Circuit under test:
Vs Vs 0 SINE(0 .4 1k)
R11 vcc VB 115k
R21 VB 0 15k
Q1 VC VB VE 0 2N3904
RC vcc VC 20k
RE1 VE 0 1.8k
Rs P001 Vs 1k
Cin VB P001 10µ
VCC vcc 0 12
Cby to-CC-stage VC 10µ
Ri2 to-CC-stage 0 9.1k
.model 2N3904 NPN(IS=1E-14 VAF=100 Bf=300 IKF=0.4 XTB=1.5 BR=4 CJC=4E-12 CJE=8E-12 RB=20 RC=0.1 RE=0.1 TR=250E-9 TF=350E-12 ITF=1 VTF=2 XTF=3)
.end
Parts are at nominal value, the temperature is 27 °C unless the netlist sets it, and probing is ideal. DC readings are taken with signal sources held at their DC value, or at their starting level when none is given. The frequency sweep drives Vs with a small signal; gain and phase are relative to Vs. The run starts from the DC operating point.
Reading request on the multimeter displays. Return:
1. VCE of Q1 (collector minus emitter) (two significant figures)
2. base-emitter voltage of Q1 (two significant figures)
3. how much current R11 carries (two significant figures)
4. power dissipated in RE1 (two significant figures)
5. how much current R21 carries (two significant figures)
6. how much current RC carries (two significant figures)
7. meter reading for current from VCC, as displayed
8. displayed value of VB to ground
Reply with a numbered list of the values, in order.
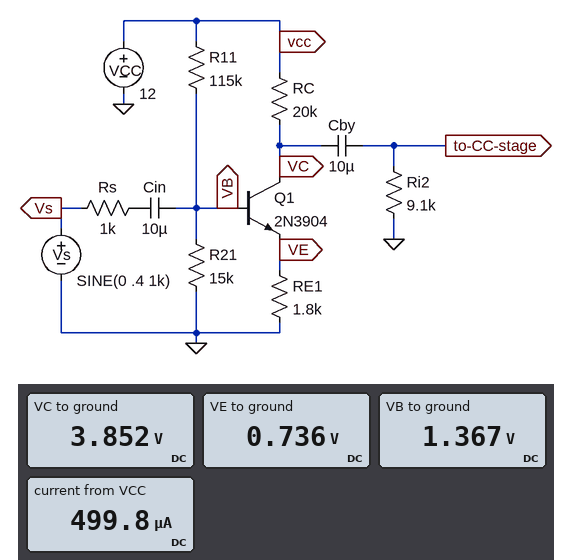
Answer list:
1. 3.1 V
2. 630 mV
3. 92 µA
4. 300 µW
5. 91 µA
6. 410 µA
7. 499.8 µA
8. 1.367 V
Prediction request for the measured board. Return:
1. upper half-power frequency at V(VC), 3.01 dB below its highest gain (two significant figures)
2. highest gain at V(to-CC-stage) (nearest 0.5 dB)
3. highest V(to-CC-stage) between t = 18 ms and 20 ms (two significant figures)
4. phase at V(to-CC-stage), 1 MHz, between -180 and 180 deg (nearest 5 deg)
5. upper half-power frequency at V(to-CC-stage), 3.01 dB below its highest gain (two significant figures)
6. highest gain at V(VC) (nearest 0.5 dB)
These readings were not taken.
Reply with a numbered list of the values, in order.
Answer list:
1. 4.3 MHz
2. 10.0 dB
3. 1.2 V
4. 170 deg
5. 6.4 MHz
6. 11.0 dB
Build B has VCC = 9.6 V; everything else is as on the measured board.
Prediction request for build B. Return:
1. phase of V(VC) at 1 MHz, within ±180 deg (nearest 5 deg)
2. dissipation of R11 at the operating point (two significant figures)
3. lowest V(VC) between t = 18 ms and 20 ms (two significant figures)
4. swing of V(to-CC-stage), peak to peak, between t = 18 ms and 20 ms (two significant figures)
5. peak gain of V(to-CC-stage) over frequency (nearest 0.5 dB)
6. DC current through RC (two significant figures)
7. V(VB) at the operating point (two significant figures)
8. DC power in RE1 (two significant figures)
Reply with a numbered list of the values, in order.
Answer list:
1. 170 deg
2. 630 µW
3. 3.1 V
4. 2.4 V
5. 9.5 dB
6. 260 µA
7. 1.1 V
8. 130 µW
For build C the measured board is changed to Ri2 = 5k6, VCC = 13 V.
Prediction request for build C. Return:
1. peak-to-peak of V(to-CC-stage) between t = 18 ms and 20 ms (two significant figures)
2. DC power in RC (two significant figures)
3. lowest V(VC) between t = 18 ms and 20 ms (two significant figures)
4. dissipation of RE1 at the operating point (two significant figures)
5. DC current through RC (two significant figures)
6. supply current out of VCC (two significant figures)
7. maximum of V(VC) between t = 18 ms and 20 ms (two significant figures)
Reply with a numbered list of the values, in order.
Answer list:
1. 1.7 V
2. 4.4 mW
3. 2.8 V
4. 400 µW
5. 470 µA
6. 570 µA
7. 4.5 V
